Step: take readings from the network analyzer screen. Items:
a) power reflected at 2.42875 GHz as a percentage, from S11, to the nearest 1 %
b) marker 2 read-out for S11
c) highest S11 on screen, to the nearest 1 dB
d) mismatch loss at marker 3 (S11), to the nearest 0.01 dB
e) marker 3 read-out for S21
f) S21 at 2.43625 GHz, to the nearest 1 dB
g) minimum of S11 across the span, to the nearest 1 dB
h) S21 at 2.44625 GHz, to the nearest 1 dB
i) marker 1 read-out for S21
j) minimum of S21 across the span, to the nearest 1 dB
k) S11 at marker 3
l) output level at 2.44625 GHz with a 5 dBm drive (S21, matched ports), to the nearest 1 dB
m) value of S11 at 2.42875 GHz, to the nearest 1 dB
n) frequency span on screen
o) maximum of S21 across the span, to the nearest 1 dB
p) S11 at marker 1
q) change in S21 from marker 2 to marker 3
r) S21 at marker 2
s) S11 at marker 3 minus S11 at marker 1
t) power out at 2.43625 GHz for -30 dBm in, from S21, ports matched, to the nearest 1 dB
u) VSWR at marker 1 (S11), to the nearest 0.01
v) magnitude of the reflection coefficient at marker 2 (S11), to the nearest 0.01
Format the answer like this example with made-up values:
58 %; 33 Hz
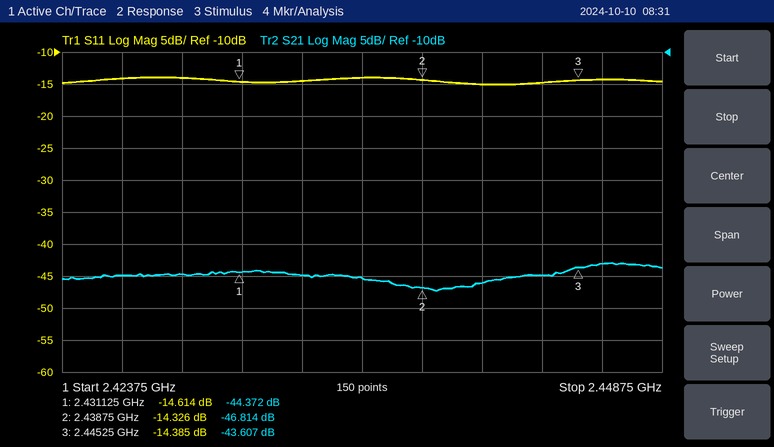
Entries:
4 %; -14.326 dB; -14 dB; 0.16 dB; -43.607 dB; -45 dB; -15 dB; -43 dB; -44.372 dB; -47 dB; -14.385 dB; -38 dBm; -14 dB; 25 MHz; -43 dB; -14.614 dB; 3.207 dB; -46.814 dB; 0.229 dB; -75 dBm; 1.46; 0.19
